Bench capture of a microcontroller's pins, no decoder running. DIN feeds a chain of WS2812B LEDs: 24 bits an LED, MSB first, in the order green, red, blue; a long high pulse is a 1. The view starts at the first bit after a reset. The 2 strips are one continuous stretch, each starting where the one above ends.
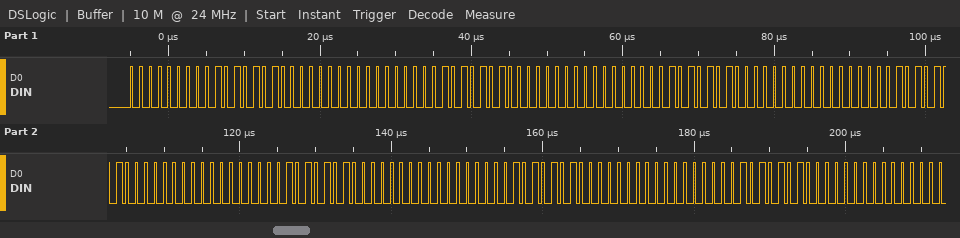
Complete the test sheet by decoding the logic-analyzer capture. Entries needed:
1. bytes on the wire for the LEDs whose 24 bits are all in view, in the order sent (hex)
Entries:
00 55 00 00 55 00 00 55 00 00 55 00 00 55 00 00 55 00 00 55 00
